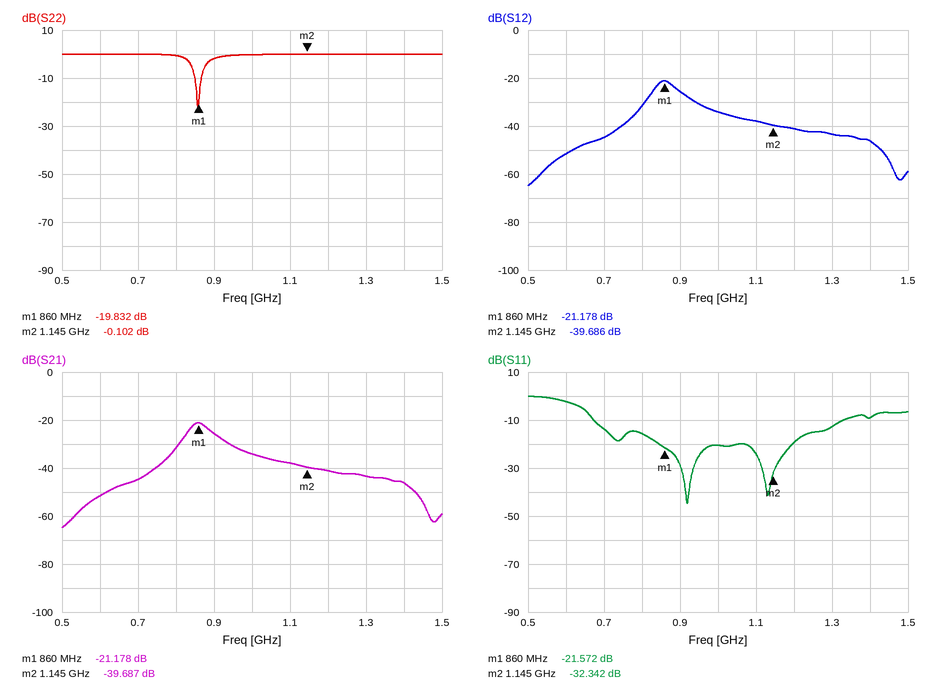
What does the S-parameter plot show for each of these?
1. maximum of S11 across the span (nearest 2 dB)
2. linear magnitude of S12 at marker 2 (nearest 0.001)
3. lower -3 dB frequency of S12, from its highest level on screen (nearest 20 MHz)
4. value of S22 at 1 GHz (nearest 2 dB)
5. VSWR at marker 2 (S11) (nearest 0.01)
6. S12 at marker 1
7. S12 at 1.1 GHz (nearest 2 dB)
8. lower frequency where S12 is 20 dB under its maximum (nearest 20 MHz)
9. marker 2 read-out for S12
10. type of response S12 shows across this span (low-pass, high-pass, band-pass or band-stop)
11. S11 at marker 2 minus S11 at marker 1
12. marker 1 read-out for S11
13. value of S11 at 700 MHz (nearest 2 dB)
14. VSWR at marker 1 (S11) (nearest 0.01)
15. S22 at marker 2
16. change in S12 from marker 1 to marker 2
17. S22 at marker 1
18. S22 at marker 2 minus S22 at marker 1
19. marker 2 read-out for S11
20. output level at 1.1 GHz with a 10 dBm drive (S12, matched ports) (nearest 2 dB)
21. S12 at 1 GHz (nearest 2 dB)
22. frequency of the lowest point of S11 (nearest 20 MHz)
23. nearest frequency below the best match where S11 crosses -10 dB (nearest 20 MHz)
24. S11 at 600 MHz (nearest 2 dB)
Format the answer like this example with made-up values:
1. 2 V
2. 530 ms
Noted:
1. 0 dB
2. 0.010
3. 840 MHz
4. 0 dB
5. 1.05
6. -21.178 dB
7. -38 dB
8. 740 MHz
9. -39.686 dB
10. band-pass
11. -10.770 dB
12. -21.572 dB
13. -14 dB
14. 1.18
15. -0.102 dB
16. -18.508 dB
17. -19.832 dB
18. 19.730 dB
19. -32.342 dB
20. -28 dBm
21. -34 dB
22. 920 MHz
23. 680 MHz
24. -2 dB
